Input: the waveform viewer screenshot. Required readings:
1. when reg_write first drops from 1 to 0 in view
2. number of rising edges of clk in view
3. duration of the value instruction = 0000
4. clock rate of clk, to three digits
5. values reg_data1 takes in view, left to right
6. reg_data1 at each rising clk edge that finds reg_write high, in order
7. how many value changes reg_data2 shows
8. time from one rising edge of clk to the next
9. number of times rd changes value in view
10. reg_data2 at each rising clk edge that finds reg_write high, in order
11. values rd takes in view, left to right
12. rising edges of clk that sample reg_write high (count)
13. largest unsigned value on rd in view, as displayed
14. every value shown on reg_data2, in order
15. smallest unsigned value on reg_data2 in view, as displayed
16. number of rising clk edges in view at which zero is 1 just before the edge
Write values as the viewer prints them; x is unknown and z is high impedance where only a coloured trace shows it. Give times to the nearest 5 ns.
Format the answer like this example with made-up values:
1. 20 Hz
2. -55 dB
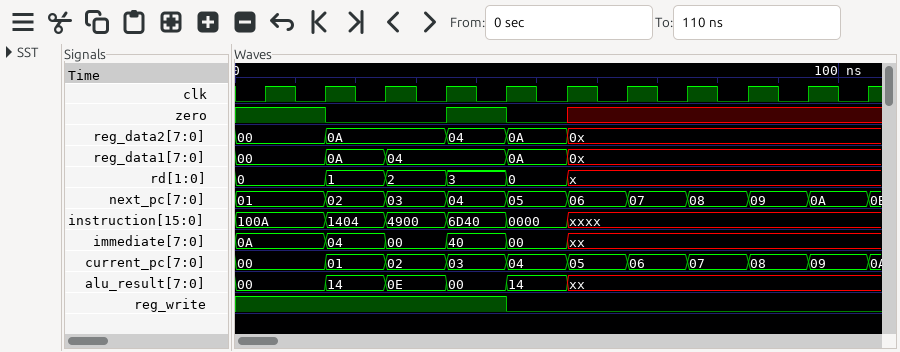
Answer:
1. 45 ns
2. 11
3. 10 ns
4. 100 MHz
5. 00, 0A, 04, 0A, 0x
6. 00, 00, 0A, 04, 04
7. 4
8. 10 ns
9. 5
10. 00, 00, 0A, 0A, 04
11. 0, 1, 2, 3, 0, x
12. 5
13. 3
14. 00, 0A, 04, 0A, 0x
15. 00
16. 3
